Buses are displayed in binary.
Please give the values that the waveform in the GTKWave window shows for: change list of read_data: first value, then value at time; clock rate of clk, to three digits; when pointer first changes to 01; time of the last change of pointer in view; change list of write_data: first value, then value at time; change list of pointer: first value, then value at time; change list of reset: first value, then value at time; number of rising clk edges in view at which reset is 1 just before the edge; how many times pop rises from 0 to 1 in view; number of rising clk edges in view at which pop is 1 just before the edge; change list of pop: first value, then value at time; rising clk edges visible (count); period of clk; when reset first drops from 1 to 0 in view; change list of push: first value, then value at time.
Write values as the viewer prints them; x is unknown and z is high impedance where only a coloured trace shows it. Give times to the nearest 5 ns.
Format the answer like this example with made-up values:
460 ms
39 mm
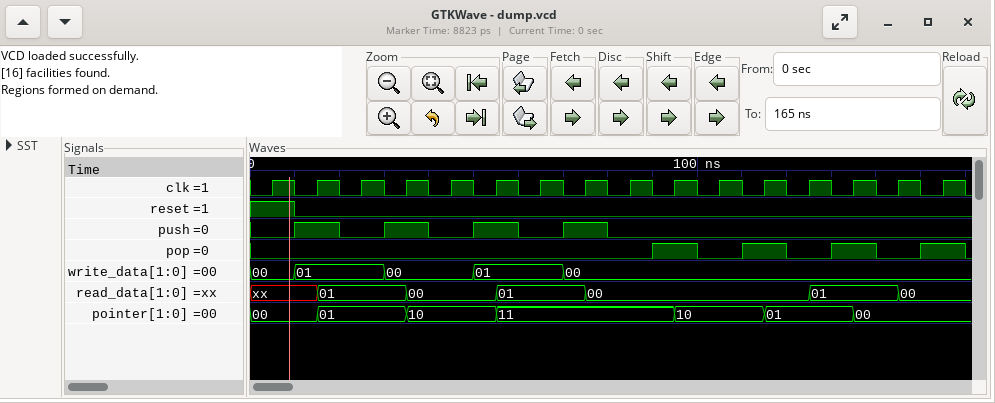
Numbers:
xx, 01 at 15 ns, 00 at 35 ns, 01 at 55 ns, 00 at 75 ns, 01 at 125 ns, 00 at 145 ns
100 MHz
15 ns
135 ns
00, 01 at 10 ns, 00 at 30 ns, 01 at 50 ns, 00 at 70 ns
00, 01 at 15 ns, 10 at 35 ns, 11 at 55 ns, 10 at 95 ns, 01 at 115 ns, 00 at 135 ns
1, 0 at 10 ns
1
4
4
0, 1 at 90 ns, 0 at 100 ns, 1 at 110 ns, 0 at 120 ns, 1 at 130 ns, 0 at 140 ns, 1 at 150 ns, 0 at 160 ns
16
10 ns
10 ns
0, 1 at 10 ns, 0 at 20 ns, 1 at 30 ns, 0 at 40 ns, 1 at 50 ns, 0 at 60 ns, 1 at 70 ns, 0 at 80 ns
